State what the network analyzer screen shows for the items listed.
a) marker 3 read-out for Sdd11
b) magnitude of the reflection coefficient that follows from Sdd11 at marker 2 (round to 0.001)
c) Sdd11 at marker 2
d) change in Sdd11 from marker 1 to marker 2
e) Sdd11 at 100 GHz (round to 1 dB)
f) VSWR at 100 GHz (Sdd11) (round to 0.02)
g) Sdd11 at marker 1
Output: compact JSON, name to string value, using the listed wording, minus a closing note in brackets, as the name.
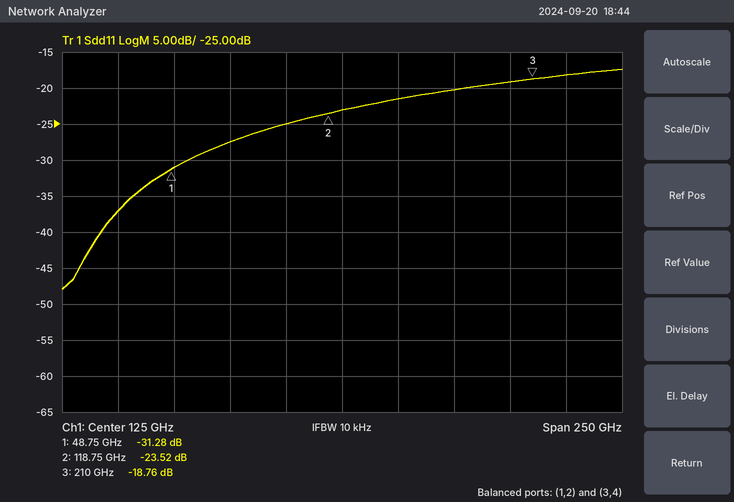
{"marker 3 read-out for Sdd11": "-18.76 dB", "magnitude of the reflection coefficient that follows from Sdd11 at marker 2": "0.067", "Sdd11 at marker 2": "-23.52 dB", "change in Sdd11 from marker 1 to marker 2": "7.76 dB", "Sdd11 at 100 GHz": "-25 dB", "VSWR at 100 GHz (Sdd11)": "1.12", "Sdd11 at marker 1": "-31.28 dB"}
